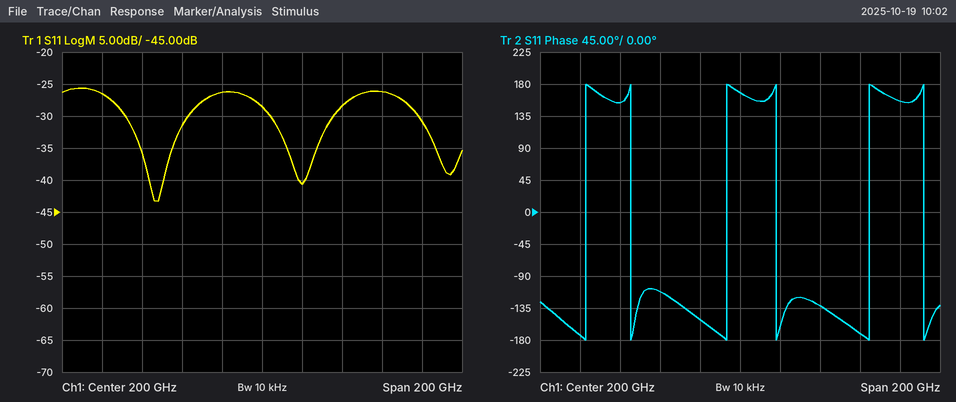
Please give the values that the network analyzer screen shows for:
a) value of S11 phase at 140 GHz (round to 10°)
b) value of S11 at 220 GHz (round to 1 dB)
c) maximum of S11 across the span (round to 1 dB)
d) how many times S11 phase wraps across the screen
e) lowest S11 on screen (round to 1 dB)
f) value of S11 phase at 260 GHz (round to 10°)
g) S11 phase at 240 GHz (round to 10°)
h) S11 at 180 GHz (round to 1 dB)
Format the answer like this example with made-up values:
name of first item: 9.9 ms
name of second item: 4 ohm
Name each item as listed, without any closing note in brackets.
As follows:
value of S11 phase at 140 GHz: 150°
value of S11 at 220 GHz: -41 dB
maximum of S11 across the span: -26 dB
how many times S11 phase wraps across the screen: 6
lowest S11 on screen: -43 dB
value of S11 phase at 260 GHz: -170°
S11 phase at 240 GHz: -130°
S11 at 180 GHz: -26 dB
